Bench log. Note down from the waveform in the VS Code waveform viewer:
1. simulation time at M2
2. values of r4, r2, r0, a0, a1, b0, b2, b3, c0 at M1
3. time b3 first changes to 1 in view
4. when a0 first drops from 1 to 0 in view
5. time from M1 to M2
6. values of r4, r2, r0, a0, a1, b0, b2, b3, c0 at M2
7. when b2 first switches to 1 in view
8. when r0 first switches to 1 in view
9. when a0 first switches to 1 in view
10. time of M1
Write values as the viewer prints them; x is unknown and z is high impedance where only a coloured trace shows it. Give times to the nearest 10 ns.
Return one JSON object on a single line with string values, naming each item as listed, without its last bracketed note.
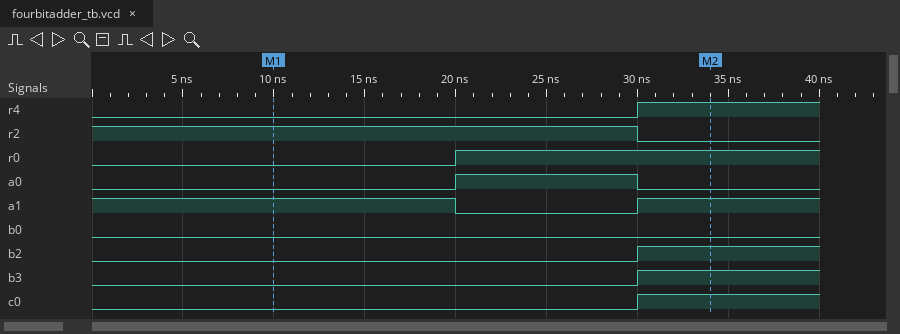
{"simulation time at M2": "30 ns", "values of r4, r2, r0, a0, a1, b0, b2, b3, c0 at M1": "r4=0, r2=1, r0=0, a0=0, a1=1, b0=0, b2=0, b3=0, c0=0", "time b3 first changes to 1 in view": "30 ns", "when a0 first drops from 1 to 0 in view": "30 ns", "time from M1 to M2": "20 ns", "values of r4, r2, r0, a0, a1, b0, b2, b3, c0 at M2": "r4=1, r2=0, r0=1, a0=0, a1=1, b0=0, b2=1, b3=1, c0=1", "when b2 first switches to 1 in view": "30 ns", "when r0 first switches to 1 in view": "20 ns", "when a0 first switches to 1 in view": "20 ns", "time of M1": "10 ns"}
